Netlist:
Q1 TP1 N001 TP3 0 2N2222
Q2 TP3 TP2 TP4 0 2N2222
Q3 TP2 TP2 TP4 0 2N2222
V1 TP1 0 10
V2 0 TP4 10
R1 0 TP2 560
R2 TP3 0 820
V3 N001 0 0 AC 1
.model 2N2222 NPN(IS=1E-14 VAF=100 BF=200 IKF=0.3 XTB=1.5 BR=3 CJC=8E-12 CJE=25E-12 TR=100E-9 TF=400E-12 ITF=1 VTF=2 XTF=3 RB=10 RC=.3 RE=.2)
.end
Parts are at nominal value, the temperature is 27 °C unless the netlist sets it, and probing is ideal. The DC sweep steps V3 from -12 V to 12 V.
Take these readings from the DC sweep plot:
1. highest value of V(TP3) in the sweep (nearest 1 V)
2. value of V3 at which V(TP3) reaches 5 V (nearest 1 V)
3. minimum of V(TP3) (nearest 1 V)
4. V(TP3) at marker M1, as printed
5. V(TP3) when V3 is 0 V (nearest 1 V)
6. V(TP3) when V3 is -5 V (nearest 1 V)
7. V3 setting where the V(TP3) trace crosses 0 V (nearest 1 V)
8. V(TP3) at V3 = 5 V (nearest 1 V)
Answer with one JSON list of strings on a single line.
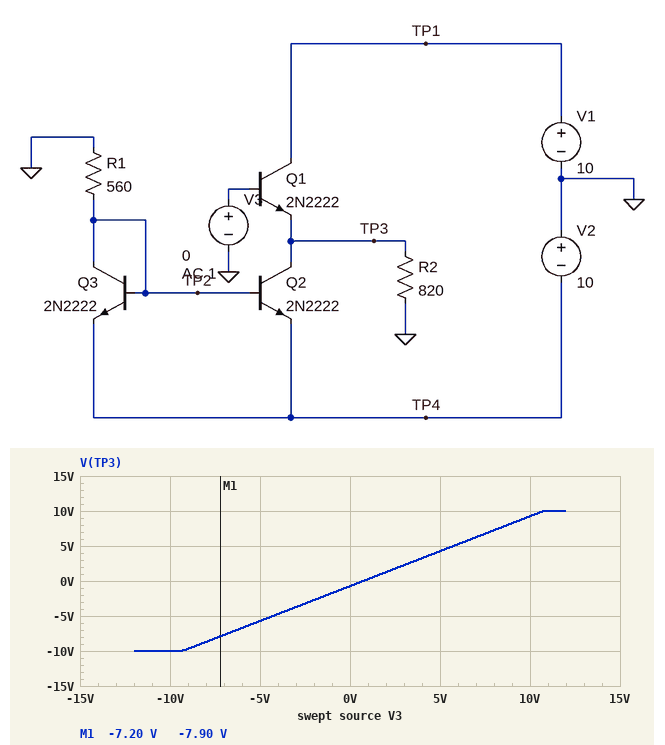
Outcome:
["10 V", "6 V", "-10 V", "-7.90 V", "-1 V", "-6 V", "1 V", "4 V"]
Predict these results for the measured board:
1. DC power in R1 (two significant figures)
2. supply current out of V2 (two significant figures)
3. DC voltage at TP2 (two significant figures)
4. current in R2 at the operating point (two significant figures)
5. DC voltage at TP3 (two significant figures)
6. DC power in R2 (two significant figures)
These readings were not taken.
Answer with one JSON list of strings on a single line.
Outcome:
["150 mW", "34 mA", "-9.3 V", "890 µA", "-730 mV", "650 µW"]
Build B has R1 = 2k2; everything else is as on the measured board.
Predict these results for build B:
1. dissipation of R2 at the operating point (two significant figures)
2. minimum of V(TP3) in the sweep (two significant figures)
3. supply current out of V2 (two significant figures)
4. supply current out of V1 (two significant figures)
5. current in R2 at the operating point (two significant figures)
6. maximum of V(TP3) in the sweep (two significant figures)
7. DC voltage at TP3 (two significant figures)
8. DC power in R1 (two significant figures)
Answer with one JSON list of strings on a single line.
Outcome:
["580 µW", "-3.6 V", "8.8 mA", "3.7 mA", "840 µA", "10 V", "-690 mV", "39 mW"]
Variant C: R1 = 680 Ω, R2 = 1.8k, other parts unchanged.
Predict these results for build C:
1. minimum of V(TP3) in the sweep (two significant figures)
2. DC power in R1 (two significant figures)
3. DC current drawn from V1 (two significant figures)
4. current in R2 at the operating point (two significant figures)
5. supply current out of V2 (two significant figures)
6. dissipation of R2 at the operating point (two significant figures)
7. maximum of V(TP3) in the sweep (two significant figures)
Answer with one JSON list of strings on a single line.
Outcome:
["-10 V", "130 mW", "14 mA", "400 µA", "28 mA", "290 µW", "10 V"]
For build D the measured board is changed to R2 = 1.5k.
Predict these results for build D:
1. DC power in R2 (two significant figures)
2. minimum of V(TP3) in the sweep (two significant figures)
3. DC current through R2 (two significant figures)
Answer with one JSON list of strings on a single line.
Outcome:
["360 µW", "-10 V", "490 µA"]
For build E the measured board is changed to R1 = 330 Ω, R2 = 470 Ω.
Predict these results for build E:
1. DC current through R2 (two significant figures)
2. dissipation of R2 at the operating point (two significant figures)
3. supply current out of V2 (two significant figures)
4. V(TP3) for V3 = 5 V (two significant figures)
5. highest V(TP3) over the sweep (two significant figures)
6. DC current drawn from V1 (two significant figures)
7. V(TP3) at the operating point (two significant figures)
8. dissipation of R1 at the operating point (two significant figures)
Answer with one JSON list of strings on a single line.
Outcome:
["1.6 mA", "1.2 mW", "58 mA", "4.2 V", "10 V", "28 mA", "-750 mV", "260 mW"]
